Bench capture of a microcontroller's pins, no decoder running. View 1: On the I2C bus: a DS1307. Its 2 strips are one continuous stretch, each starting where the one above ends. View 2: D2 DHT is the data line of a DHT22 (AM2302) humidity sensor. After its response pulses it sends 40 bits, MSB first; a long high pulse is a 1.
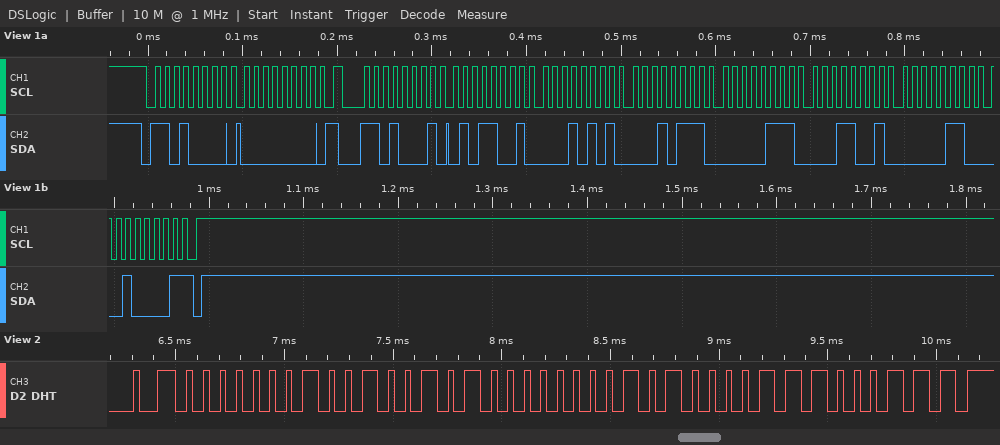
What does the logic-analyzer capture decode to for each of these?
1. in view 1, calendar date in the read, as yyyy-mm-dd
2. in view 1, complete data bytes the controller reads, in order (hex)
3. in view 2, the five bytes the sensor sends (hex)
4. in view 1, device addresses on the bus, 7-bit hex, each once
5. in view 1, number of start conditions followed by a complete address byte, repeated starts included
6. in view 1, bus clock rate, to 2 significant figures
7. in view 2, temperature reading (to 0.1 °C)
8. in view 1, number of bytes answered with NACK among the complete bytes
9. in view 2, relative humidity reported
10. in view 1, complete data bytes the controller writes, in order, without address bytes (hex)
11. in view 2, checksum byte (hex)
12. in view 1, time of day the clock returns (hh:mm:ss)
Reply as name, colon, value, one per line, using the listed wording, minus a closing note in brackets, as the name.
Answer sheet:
in view 1, calendar date in the read, as yyyy-mm-dd: 2021-06-19
in view 1, complete data bytes the controller reads, in order: 59 15 17 07 19 06 21
in view 2, the five bytes the sensor sends: 01 25 00 A1 C7
in view 1, device addresses on the bus, 7-bit hex, each once: 0x68
in view 1, number of start conditions followed by a complete address byte, repeated starts included: 2
in view 1, bus clock rate, to 2 significant figures: 100 kHz
in view 2, temperature reading: 16.1 °C
in view 1, number of bytes answered with NACK among the complete bytes: 1
in view 2, relative humidity reported: 29.3 %
in view 1, complete data bytes the controller writes, in order, without address bytes: 00
in view 2, checksum byte: 0xC7
in view 1, time of day the clock returns: 17:15:59
